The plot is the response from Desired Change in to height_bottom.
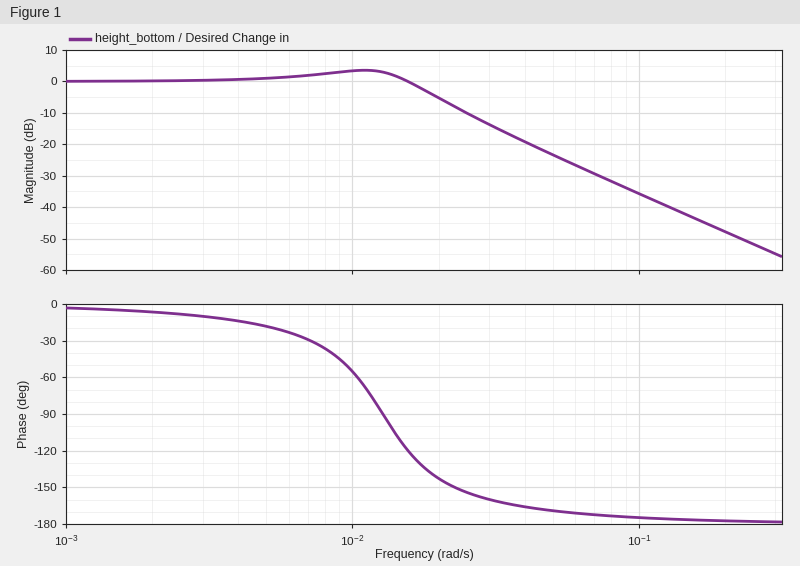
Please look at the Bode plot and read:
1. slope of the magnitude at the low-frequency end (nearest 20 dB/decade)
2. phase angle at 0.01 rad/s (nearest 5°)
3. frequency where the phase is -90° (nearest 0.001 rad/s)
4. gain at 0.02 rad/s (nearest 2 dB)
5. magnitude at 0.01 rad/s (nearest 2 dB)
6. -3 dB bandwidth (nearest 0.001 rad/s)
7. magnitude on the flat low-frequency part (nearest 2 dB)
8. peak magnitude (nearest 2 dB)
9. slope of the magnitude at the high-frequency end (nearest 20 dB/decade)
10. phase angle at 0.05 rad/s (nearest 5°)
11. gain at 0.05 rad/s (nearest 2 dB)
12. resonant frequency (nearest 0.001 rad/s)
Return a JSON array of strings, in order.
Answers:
["0 dB/decade", "-55°", "0.013 rad/s", "-6 dB", "4 dB", "0.018 rad/s", "0 dB", "4 dB", "-40 dB/decade", "-170°", "-24 dB", "0.011 rad/s"]
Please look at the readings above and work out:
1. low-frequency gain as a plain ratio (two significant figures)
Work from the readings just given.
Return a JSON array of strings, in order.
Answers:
["1.0"]
